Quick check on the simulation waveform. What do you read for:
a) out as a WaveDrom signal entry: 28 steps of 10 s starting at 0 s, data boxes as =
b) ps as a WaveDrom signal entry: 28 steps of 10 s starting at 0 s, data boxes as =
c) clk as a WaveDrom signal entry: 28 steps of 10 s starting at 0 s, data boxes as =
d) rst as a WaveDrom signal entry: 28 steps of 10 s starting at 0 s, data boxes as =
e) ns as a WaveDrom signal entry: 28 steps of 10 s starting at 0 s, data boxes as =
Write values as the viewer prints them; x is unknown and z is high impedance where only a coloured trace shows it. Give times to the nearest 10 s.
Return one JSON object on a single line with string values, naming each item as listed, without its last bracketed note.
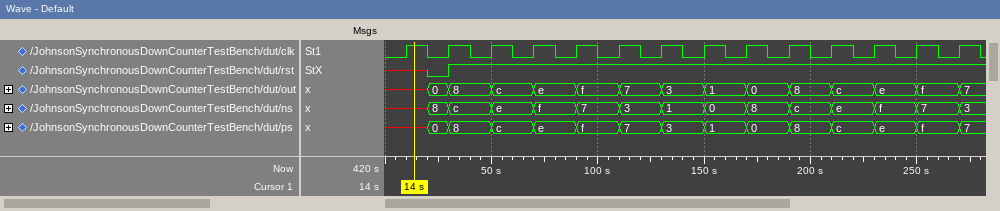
{"out as a WaveDrom signal entry: 28 steps of 10 s starting at 0 s, data boxes as =": "{name: 'out', wave: 'x.==.=.=.=.=.=.=.=.=.=.=.=.=', data: '0 8 c e f 7 3 1 0 8 c e f 7'}", "ps as a WaveDrom signal entry: 28 steps of 10 s starting at 0 s, data boxes as =": "{name: 'ps', wave: 'x.==.=.=.=.=.=.=.=.=.=.=.=.=', data: '0 8 c e f 7 3 1 0 8 c e f 7'}", "clk as a WaveDrom signal entry: 28 steps of 10 s starting at 0 s, data boxes as =": "{name: 'clk', wave: '0101010101010101010101010101'}", "rst as a WaveDrom signal entry: 28 steps of 10 s starting at 0 s, data boxes as =": "{name: 'rst', wave: 'x.01........................'}", "ns as a WaveDrom signal entry: 28 steps of 10 s starting at 0 s, data boxes as =": "{name: 'ns', wave: 'x.==.=.=.=.=.=.=.=.=.=.=.=.=', data: '8 c e f 7 3 1 0 8 c e f 7 3'}"}
